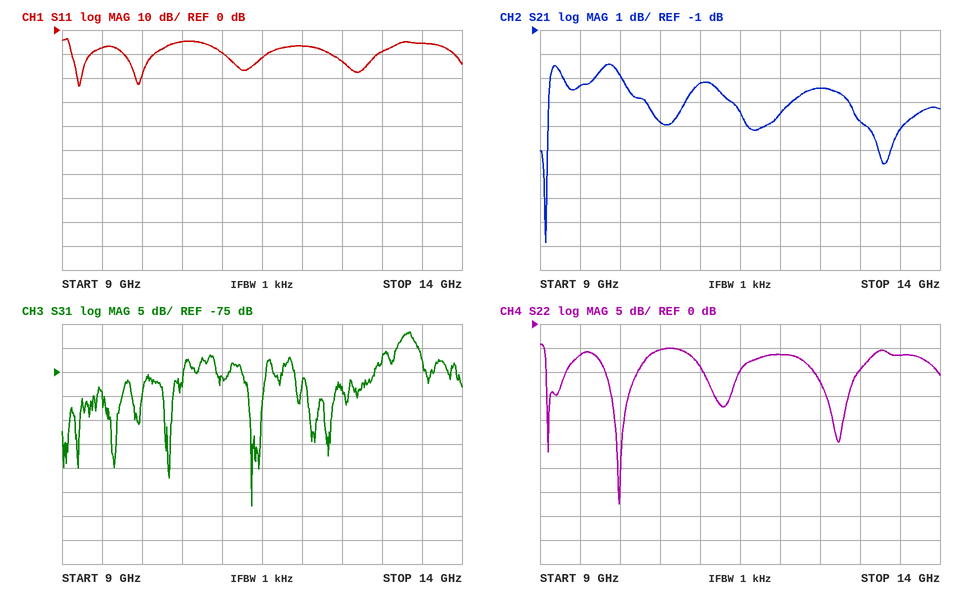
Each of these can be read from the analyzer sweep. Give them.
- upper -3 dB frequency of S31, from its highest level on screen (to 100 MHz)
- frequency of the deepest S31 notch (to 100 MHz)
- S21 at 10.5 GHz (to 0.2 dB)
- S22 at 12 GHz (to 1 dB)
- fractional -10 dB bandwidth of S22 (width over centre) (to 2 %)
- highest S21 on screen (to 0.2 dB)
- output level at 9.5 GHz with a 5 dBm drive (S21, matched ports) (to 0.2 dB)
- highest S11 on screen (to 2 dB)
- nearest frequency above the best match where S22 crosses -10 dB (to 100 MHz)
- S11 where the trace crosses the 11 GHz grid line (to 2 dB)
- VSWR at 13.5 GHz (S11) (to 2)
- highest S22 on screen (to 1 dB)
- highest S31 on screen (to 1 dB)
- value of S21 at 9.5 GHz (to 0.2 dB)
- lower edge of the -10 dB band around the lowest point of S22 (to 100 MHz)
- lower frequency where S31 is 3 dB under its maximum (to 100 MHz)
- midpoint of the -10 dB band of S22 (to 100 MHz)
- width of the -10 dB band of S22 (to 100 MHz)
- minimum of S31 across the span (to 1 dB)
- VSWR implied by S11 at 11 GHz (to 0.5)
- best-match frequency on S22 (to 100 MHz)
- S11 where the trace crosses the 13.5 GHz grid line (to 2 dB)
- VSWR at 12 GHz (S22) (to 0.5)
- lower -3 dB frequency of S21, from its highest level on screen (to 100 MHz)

13.4 GHz
11.4 GHz
-4.8 dB
-6 dB
4 %
-2.4 dB
1.6 dBm
-4 dB
10.2 GHz
-10 dB
4
-4 dB
-67 dB
-3.4 dB
9.8 GHz
13.2 GHz
10.0 GHz
400 MHz
-103 dB
2.0
10.0 GHz
-6 dB
3.0
9.1 GHz
